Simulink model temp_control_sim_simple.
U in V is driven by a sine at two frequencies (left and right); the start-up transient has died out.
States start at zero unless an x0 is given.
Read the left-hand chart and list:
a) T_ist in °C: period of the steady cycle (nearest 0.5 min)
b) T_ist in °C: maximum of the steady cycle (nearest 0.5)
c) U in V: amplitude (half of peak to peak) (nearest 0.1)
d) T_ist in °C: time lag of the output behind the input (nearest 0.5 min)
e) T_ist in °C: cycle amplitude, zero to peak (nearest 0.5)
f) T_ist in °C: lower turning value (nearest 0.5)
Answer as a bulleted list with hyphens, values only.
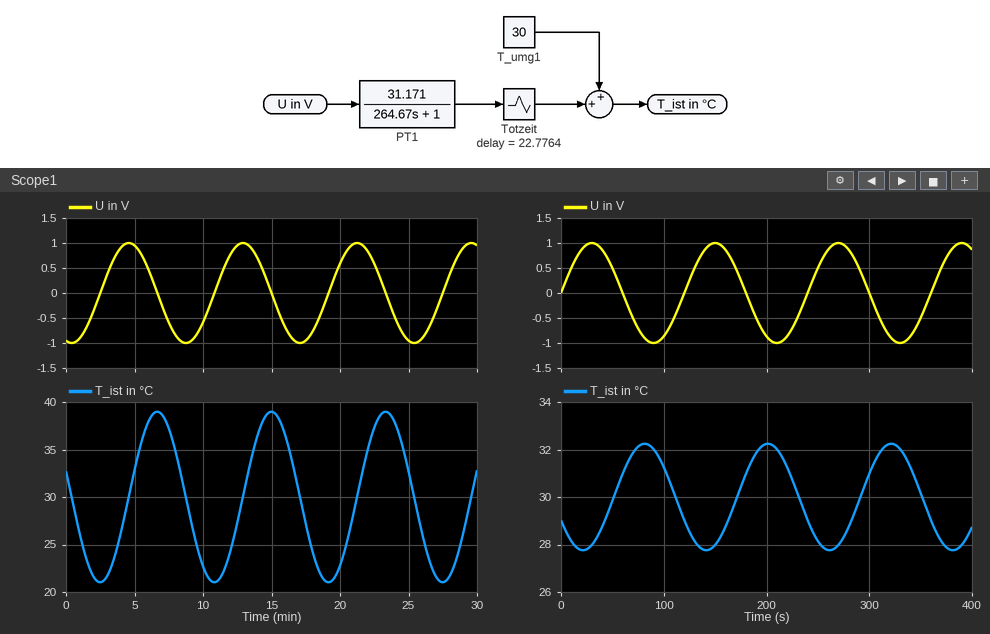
- 8.5 min
- 39.0
- 1.0
- 2.0 min
- 9.0
- 21.0
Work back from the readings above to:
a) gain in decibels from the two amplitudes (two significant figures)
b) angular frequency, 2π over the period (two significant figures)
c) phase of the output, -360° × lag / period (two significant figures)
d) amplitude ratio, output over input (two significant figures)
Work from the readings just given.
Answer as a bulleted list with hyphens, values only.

- 19 dB
- 0.74 rad/min
- -85°
- 9.0
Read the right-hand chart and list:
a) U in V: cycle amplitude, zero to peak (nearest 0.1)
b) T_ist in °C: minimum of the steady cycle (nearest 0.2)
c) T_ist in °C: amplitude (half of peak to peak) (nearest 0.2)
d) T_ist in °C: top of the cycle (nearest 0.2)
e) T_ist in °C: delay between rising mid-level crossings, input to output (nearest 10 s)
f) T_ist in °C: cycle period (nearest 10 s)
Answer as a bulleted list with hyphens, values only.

- 1.0
- 27.8
- 2.2
- 32.2
- 50 s
- 120 s
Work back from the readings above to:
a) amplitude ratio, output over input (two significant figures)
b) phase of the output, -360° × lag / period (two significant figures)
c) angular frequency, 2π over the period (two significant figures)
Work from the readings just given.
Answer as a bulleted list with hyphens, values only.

- 2.2
- -150°
- 0.052 rad/s
